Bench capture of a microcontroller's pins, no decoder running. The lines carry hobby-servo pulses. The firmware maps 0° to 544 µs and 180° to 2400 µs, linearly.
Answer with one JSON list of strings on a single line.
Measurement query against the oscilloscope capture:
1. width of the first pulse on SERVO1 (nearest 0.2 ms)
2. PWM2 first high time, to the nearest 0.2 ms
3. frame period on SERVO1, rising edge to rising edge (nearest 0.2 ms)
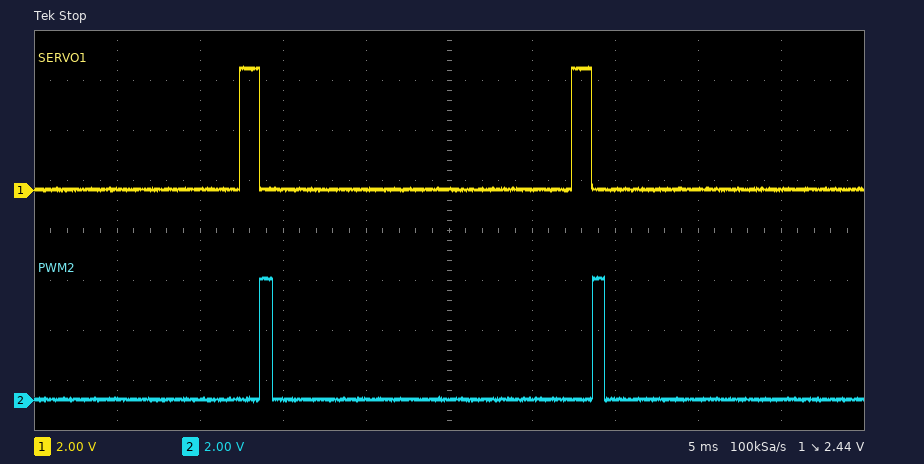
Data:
["1.2 ms", "0.8 ms", "20.0 ms"]
